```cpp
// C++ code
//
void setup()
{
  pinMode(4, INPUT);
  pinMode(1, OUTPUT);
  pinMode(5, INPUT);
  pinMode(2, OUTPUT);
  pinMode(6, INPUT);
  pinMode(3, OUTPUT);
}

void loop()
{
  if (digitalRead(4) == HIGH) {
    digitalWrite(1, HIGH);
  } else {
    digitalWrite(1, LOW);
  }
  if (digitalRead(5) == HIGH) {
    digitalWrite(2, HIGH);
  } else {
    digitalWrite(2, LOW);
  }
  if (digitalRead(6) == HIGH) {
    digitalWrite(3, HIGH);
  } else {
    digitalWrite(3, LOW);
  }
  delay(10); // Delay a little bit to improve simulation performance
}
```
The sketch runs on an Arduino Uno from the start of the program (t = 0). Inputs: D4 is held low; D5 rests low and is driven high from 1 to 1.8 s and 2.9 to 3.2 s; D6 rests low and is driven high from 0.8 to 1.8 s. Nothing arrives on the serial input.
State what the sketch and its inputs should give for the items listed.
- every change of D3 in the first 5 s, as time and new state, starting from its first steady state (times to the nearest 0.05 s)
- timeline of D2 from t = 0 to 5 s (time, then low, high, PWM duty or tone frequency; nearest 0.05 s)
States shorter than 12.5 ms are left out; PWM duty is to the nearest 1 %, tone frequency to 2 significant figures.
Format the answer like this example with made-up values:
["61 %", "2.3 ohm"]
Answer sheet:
["0 s low; 0.8 s high; 1.8 s low", "0 s low; 1 s high; 1.8 s low; 2.9 s high; 3.2 s low"]
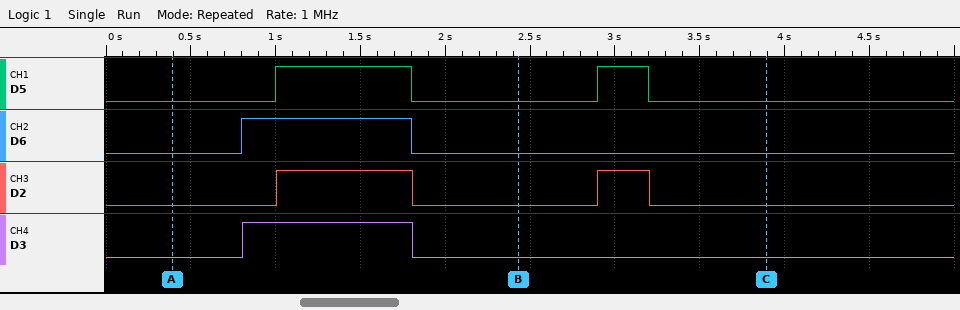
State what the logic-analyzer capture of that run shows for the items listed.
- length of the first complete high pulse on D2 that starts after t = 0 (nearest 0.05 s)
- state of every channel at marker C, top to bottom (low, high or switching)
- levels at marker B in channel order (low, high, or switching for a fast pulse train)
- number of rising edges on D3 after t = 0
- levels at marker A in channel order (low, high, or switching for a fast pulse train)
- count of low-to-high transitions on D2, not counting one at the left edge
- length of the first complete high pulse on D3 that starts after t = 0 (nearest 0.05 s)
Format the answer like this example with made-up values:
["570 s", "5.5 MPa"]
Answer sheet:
["0.80 s", "D5 low, D6 low, D2 low, D3 low", "D5 low, D6 low, D2 low, D3 low", "1", "D5 low, D6 low, D2 low, D3 low", "2", "1.00 s"]
